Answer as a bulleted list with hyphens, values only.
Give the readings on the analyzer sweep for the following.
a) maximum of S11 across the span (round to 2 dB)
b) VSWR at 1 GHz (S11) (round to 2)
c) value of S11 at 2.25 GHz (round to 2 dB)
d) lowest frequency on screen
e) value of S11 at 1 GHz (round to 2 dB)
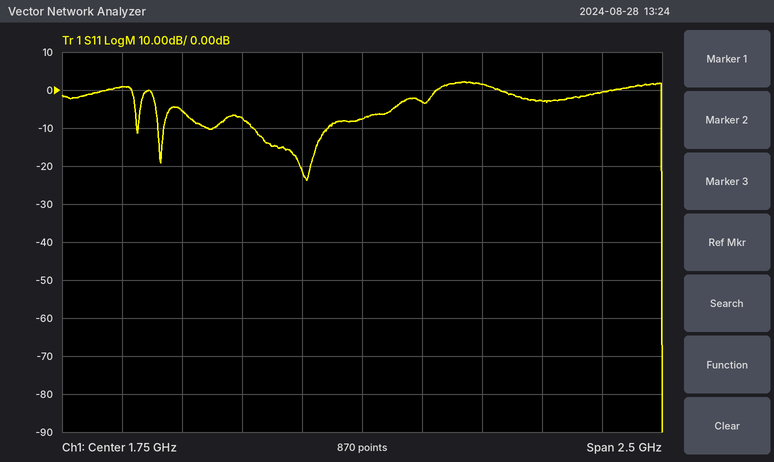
- 2 dB
- 4
- 2 dB
- 500 MHz
- -6 dB
